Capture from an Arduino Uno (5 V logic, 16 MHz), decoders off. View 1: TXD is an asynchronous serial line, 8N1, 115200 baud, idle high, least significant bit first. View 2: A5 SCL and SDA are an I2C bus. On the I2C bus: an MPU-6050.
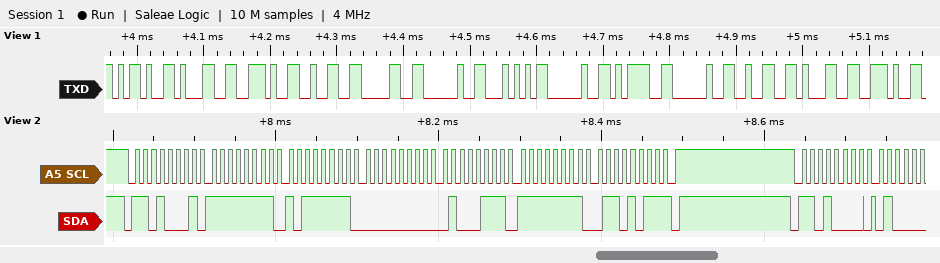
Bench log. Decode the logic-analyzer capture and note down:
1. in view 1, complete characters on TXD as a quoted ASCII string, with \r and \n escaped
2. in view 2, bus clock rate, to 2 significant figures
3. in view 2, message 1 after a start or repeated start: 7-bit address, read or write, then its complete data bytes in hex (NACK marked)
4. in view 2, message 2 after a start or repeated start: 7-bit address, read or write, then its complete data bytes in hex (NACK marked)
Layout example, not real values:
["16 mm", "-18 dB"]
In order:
["\"-1.20 T = 21.\"", "100 kHz", "0x68 read: FF BF 00 47 FF 6B NACK", "0x68 write"]
